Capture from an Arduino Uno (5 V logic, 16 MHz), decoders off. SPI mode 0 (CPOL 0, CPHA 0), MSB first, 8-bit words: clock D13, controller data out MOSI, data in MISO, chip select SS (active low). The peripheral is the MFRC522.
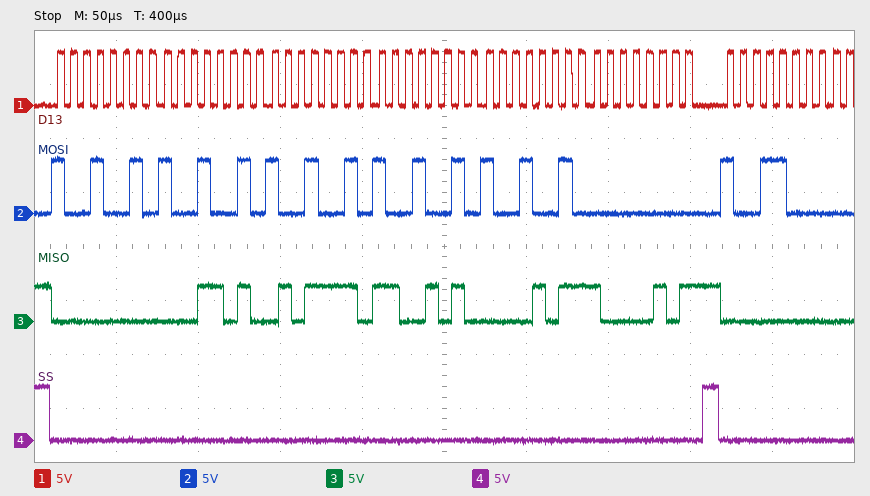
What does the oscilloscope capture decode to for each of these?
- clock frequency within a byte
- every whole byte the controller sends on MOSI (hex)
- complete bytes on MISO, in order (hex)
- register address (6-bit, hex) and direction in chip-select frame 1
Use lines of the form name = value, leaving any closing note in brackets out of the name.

clock frequency within a byte = 125 kHz
every whole byte the controller sends on MOSI = 0x92 0x92 0x92 0x92 0x92 0x00 0x98
complete bytes on MISO, in order = 0x00 0x1A 0x5E 0xCA 0x0B 0x85 0x00
register address (6-bit, hex) and direction in chip-select frame 1 = 0x09 read
